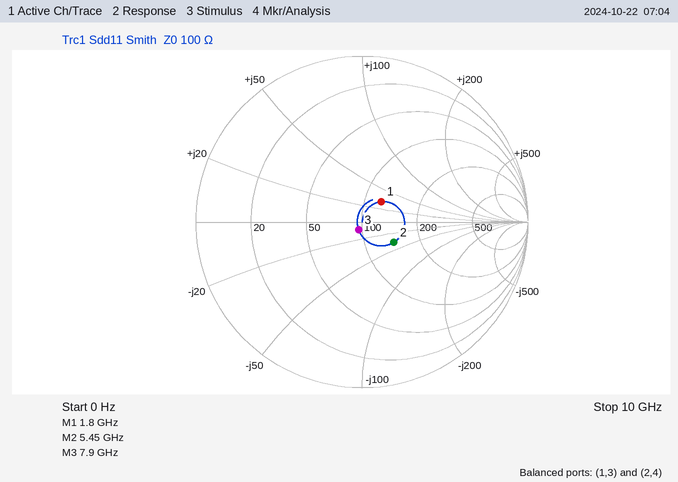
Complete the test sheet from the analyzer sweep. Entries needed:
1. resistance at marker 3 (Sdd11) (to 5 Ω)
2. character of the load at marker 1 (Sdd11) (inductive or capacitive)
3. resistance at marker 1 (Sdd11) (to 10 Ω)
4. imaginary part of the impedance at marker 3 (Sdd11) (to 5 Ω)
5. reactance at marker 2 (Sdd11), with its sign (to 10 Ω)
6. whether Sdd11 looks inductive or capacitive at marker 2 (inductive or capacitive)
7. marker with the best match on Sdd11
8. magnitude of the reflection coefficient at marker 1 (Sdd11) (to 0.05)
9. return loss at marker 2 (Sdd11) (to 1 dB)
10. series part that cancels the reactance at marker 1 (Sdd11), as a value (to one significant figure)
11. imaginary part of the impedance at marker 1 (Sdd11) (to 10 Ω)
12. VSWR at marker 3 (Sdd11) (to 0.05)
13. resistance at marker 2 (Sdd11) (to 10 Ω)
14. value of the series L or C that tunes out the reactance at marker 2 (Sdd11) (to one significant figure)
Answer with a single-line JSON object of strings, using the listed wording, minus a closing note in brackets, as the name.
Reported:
{"resistance at marker 3 (Sdd11)": "95 Ω", "character of the load at marker 1 (Sdd11)": "inductive", "resistance at marker 1 (Sdd11)": "120 Ω", "imaginary part of the impedance at marker 3 (Sdd11)": "-10 Ω", "reactance at marker 2 (Sdd11), with its sign": "-40 Ω", "whether Sdd11 looks inductive or capacitive at marker 2": "capacitive", "marker with the best match on Sdd11": "marker 3", "magnitude of the reflection coefficient at marker 1 (Sdd11)": "0.15", "return loss at marker 2 (Sdd11)": "13 dB", "series part that cancels the reactance at marker 1 (Sdd11), as a value": "3 pF", "imaginary part of the impedance at marker 1 (Sdd11)": "+30 Ω", "VSWR at marker 3 (Sdd11)": "1.10", "resistance at marker 2 (Sdd11)": "140 Ω", "value of the series L or C that tunes out the reactance at marker 2 (Sdd11)": "1 nH"}
